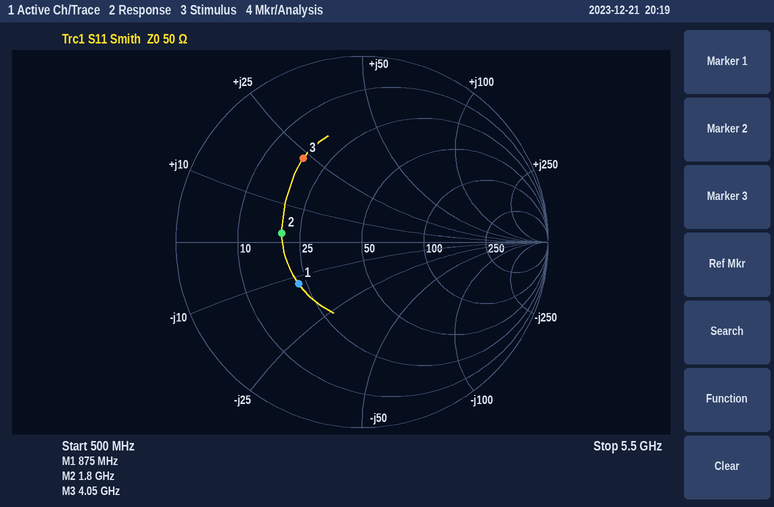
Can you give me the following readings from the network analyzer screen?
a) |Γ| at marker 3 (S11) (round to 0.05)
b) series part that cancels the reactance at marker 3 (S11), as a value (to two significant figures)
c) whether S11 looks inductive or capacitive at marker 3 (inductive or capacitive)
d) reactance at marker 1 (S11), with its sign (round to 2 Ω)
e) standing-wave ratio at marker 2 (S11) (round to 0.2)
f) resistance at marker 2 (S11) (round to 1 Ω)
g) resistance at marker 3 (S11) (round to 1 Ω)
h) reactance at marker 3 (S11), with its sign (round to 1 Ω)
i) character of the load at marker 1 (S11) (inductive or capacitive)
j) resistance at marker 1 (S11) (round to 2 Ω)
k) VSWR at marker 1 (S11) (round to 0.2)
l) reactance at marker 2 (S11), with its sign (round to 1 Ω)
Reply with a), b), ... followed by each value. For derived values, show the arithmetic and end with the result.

a) 0.55
b) C = 1/(2π × 4.05 GHz × 23 Ω) ≈ 1.7 pF
c) inductive
d) -12 Ω
e) 2.6
f) 20 Ω
g) 18 Ω
h) +23 Ω
i) capacitive
j) 22 Ω
k) 2.4
l) +2 Ω
